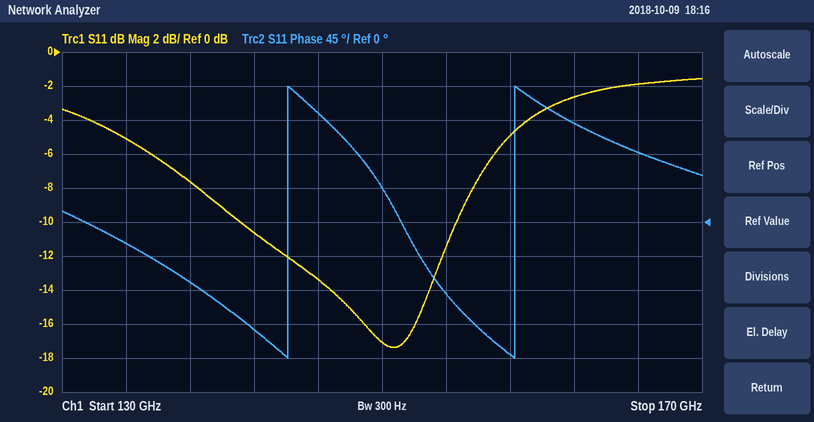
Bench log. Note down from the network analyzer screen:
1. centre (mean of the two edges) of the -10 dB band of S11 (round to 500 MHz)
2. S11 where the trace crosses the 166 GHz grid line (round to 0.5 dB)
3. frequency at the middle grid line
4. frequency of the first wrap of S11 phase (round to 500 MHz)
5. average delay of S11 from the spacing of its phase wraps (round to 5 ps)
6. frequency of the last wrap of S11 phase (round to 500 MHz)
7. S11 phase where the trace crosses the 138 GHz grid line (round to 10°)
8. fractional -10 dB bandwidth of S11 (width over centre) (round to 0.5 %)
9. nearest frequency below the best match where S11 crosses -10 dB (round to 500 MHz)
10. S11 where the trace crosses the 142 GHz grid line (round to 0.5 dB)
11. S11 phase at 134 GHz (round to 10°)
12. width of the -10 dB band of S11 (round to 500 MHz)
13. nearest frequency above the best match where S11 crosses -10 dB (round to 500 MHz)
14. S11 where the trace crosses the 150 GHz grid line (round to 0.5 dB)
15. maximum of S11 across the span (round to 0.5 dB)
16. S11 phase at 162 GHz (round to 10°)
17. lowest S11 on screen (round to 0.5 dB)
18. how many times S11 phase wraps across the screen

148.0 GHz
-2.0 dB
150 GHz
144.0 GHz
70 ps
158.5 GHz
-80°
9.0 %
141.0 GHz
-10.5 dB
-30°
13.5 GHz
154.5 GHz
-17.0 dB
-1.5 dB
130°
-17.5 dB
2
